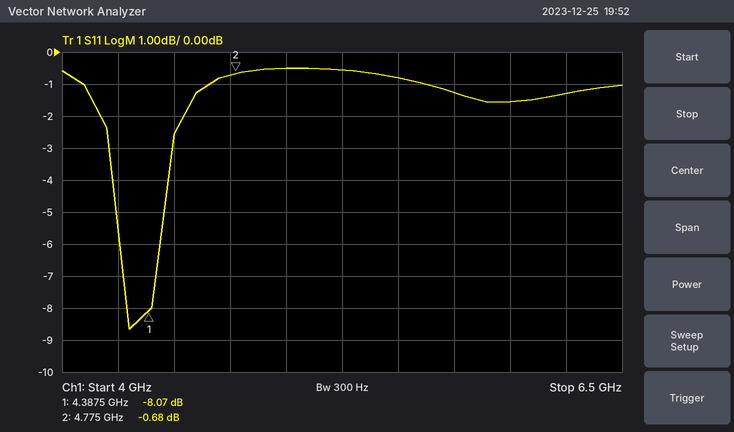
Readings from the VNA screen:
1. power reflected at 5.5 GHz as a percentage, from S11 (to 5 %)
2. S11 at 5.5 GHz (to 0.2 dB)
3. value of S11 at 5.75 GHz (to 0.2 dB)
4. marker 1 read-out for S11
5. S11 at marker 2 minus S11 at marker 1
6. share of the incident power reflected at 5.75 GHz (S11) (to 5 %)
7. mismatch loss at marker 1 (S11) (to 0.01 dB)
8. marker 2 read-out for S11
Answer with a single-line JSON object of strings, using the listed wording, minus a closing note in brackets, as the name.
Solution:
{"power reflected at 5.5 GHz as a percentage, from S11": "85 %", "S11 at 5.5 GHz": "-0.8 dB", "value of S11 at 5.75 GHz": "-1.2 dB", "marker 1 read-out for S11": "-8.07 dB", "S11 at marker 2 minus S11 at marker 1": "7.39 dB", "share of the incident power reflected at 5.75 GHz (S11)": "75 %", "mismatch loss at marker 1 (S11)": "0.74 dB", "marker 2 read-out for S11": "-0.68 dB"}
